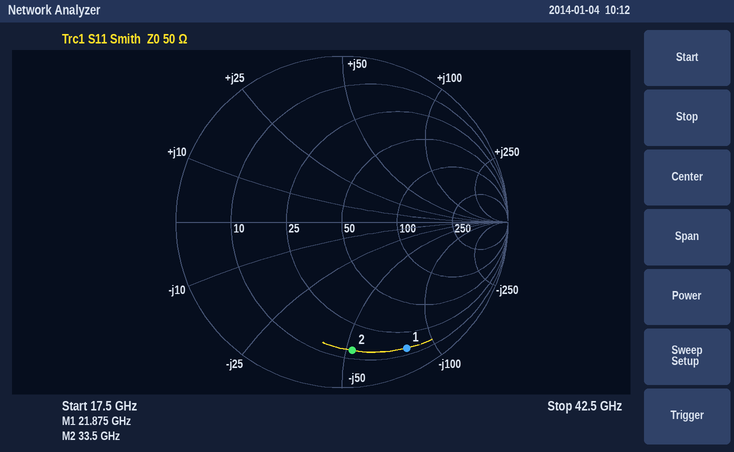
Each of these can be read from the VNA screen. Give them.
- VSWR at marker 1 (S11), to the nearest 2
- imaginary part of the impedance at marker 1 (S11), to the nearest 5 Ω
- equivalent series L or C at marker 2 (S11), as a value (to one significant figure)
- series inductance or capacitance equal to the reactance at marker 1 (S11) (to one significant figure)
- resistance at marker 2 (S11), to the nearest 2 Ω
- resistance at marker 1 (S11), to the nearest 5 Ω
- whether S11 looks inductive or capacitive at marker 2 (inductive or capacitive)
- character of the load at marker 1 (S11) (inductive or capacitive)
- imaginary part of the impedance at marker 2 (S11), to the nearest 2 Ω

12
-80 Ω
90 fF
90 fF
14 Ω
15 Ω
capacitive
capacitive
-52 Ω
